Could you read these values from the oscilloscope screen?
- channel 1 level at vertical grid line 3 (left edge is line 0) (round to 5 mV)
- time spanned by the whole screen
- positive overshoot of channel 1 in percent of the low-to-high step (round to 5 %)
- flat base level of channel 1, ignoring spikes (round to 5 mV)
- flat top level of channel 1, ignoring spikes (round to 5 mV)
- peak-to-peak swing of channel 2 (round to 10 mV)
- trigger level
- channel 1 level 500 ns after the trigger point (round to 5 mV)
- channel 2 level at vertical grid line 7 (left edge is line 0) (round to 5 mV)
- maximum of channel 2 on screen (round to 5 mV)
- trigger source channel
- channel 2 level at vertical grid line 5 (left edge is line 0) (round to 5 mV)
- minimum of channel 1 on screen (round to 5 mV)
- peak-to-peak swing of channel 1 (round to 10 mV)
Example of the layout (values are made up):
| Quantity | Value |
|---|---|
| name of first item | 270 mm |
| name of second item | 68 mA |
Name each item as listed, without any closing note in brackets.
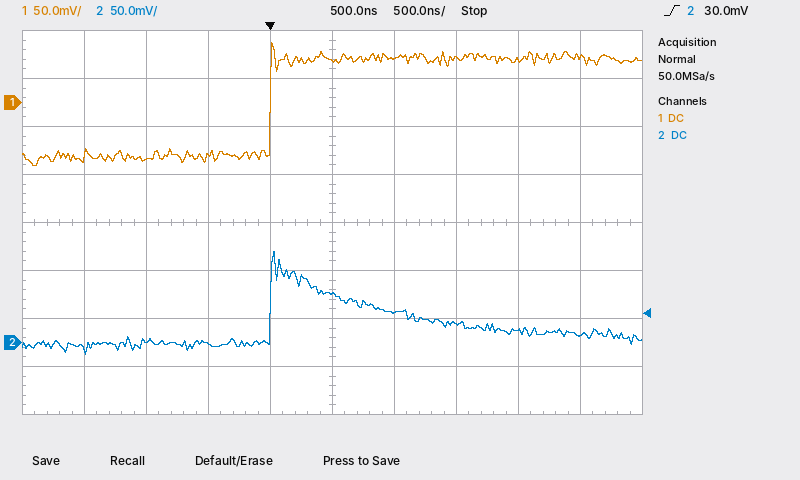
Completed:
| Quantity | Value |
|---|---|
| channel 1 level at vertical grid line 3 (left edge is line 0) | -55 mV |
| time spanned by the whole screen | 5 µs |
| positive overshoot of channel 1 in percent of the low-to-high step | 15 % |
| flat base level of channel 1, ignoring spikes | -55 mV |
| flat top level of channel 1, ignoring spikes | 45 mV |
| peak-to-peak swing of channel 2 | 110 mV |
| trigger level | 30.0 mV |
| channel 1 level 500 ns after the trigger point | 45 mV |
| channel 2 level at vertical grid line 7 (left edge is line 0) | 20 mV |
| maximum of channel 2 on screen | 95 mV |
| trigger source channel | channel 2 |
| channel 2 level at vertical grid line 5 (left edge is line 0) | 50 mV |
| minimum of channel 1 on screen | -65 mV |
| peak-to-peak swing of channel 1 | 130 mV |
